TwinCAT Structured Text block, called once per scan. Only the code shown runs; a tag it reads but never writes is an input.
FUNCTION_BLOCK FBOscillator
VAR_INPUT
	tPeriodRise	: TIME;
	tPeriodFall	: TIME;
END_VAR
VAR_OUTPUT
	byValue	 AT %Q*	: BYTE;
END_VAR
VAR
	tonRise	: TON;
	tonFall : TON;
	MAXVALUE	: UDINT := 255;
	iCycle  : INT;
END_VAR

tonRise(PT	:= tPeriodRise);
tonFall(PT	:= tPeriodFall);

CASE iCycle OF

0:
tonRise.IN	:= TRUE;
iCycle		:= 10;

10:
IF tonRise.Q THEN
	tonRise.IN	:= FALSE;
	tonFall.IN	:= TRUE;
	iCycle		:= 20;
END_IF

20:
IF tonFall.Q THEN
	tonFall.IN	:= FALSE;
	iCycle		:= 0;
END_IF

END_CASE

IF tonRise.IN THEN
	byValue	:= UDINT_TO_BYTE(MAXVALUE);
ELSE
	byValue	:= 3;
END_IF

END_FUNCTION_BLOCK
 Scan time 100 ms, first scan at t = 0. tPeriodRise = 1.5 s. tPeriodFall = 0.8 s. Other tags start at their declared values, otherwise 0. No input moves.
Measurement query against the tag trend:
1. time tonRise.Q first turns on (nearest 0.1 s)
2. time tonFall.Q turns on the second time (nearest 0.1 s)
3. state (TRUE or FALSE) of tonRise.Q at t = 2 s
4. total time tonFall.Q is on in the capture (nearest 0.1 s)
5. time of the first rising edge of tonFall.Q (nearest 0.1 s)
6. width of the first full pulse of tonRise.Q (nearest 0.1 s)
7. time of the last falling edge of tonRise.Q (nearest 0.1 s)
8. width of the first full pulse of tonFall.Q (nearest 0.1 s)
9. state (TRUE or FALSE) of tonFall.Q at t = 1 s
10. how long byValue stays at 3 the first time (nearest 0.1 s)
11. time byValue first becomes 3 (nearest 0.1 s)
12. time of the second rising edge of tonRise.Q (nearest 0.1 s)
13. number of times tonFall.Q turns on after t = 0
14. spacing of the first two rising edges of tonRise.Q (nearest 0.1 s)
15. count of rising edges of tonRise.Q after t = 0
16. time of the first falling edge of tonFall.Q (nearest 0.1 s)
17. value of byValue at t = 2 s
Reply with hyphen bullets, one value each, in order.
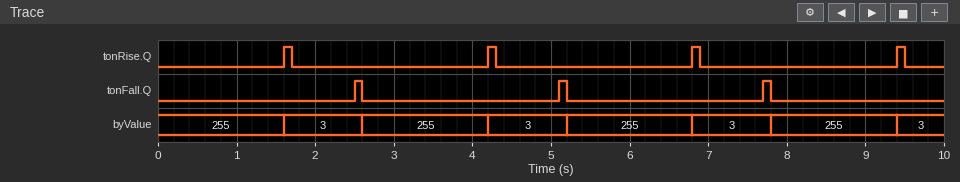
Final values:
- 1.6 s
- 5.1 s
- FALSE
- 0.3 s
- 2.5 s
- 0.1 s
- 9.5 s
- 0.1 s
- FALSE
- 1.0 s
- 1.6 s
- 4.2 s
- 3
- 2.6 s
- 4
- 2.6 s
- 3
